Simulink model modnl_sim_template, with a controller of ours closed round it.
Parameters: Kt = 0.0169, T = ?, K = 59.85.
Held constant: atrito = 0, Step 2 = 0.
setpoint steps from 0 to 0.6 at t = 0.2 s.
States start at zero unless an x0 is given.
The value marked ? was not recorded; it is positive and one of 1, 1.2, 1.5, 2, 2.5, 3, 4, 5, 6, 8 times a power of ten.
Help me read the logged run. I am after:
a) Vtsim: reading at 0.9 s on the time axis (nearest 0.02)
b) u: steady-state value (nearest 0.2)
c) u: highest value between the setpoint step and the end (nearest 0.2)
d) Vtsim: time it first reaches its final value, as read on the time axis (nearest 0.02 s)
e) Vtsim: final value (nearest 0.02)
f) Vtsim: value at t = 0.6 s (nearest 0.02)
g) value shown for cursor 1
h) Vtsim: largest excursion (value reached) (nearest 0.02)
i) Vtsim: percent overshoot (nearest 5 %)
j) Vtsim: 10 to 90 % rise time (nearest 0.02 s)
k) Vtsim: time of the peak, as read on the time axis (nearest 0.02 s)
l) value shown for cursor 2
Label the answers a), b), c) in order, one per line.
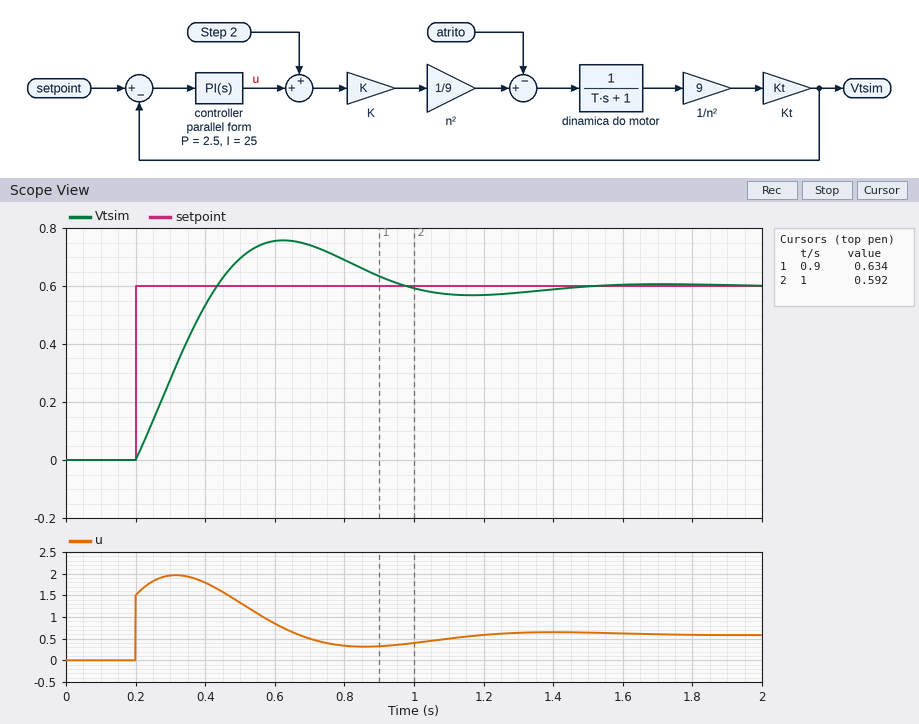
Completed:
a) 0.64
b) 0.6
c) 2.0
d) 0.44 s
e) 0.60
f) 0.76
g) 0.634
h) 0.76
i) 25 %
j) 0.18 s
k) 0.62 s
l) 0.592
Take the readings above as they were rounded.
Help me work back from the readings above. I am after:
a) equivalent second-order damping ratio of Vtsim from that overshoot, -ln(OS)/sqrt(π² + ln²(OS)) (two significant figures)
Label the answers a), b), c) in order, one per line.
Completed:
a) 0.40
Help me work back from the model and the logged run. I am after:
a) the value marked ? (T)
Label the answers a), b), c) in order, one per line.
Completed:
a) 0.6
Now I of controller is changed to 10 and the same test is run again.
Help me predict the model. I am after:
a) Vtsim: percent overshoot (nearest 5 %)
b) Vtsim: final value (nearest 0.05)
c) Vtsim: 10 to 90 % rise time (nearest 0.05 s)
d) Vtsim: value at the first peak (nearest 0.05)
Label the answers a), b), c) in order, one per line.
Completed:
a) 10 %
b) 0.60
c) 0.30 s
d) 0.65
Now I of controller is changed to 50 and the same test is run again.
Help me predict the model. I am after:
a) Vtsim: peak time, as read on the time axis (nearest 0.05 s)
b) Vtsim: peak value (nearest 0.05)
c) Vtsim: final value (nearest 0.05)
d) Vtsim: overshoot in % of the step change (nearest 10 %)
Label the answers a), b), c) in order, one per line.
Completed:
a) 0.50 s
b) 0.85
c) 0.60
d) 40 %
